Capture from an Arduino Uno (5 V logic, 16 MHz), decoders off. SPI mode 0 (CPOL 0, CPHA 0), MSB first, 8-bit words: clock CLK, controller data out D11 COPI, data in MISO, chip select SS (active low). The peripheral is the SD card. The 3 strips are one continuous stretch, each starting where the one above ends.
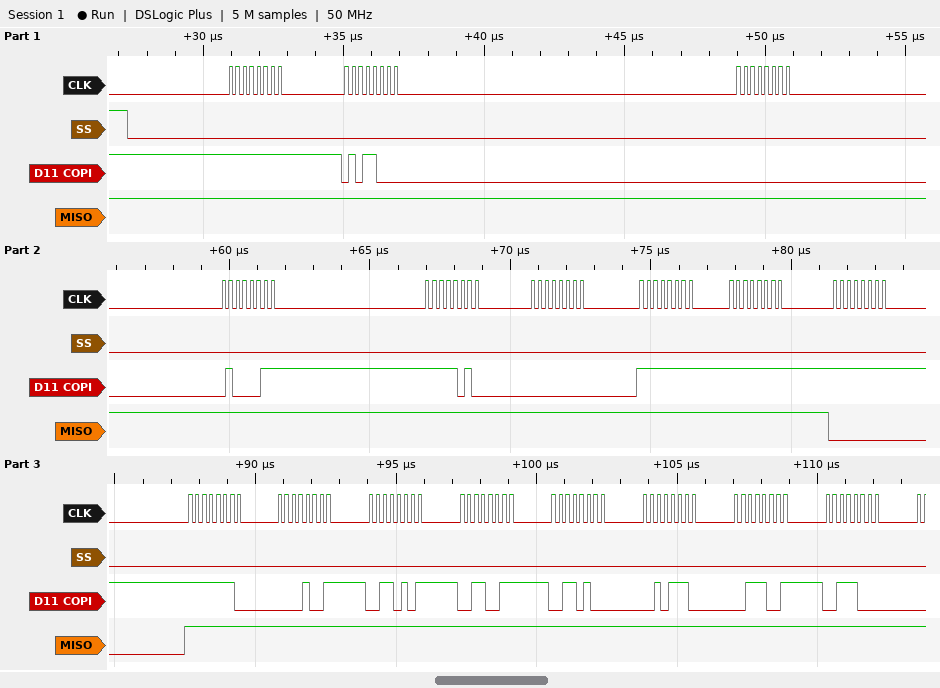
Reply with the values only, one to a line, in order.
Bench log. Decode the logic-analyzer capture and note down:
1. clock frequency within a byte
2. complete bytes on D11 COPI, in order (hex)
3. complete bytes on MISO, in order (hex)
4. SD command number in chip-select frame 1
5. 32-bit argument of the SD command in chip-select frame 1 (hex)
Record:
4 MHz
FF 58 00 43 FA 00 FF FF FF FE 09 35 33 34 2E 39 38
FF FF FF FF FF FF FF FF 00 FF FF FF FF FF FF FF FF
CMD24
0x0043FA00
